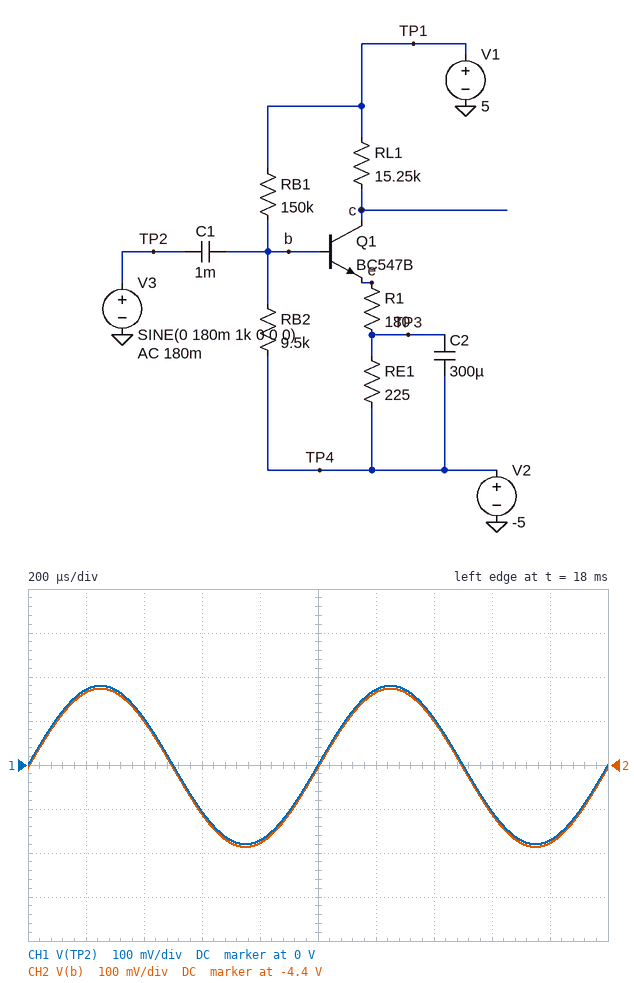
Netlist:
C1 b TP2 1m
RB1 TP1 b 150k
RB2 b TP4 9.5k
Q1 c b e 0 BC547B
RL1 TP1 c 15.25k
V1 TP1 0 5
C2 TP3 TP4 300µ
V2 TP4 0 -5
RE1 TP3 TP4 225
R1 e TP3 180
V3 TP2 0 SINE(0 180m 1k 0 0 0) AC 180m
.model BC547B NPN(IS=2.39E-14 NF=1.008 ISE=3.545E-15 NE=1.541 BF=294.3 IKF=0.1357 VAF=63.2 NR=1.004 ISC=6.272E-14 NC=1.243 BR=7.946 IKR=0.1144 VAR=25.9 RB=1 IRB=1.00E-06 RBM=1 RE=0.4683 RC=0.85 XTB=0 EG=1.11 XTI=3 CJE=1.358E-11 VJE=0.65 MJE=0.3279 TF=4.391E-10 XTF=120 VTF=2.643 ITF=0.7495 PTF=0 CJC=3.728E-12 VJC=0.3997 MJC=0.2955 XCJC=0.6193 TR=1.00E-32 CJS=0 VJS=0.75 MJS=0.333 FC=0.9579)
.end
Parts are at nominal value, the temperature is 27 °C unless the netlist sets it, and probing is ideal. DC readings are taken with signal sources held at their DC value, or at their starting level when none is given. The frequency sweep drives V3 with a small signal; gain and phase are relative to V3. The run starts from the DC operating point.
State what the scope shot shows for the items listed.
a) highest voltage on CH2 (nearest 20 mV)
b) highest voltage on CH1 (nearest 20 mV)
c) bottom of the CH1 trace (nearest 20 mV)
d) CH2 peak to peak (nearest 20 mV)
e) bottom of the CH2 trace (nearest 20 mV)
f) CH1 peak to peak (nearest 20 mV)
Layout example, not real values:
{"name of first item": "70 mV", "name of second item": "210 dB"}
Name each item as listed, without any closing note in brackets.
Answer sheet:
{"highest voltage on CH2": "-4.22 V", "highest voltage on CH1": "180 mV", "bottom of the CH1 trace": "-180 mV", "CH2 peak to peak": "360 mV", "bottom of the CH2 trace": "-4.58 V", "CH1 peak to peak": "360 mV"}
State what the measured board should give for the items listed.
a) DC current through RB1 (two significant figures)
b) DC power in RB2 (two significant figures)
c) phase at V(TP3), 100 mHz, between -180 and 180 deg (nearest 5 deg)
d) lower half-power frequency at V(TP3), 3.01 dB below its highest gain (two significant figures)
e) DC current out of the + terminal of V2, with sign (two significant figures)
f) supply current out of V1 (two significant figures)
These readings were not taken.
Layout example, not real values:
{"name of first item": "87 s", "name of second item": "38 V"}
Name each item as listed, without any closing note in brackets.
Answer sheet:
{"DC current through RB1": "63 µA", "DC power in RB2": "37 µW", "phase at V(TP3), 100 mHz, between -180 and 180 deg": "10 deg", "lower half-power frequency at V(TP3), 3.01 dB below its highest gain": "18 mHz", "DC current out of the + terminal of V2, with sign": "-130 µA", "supply current out of V1": "130 µA"}
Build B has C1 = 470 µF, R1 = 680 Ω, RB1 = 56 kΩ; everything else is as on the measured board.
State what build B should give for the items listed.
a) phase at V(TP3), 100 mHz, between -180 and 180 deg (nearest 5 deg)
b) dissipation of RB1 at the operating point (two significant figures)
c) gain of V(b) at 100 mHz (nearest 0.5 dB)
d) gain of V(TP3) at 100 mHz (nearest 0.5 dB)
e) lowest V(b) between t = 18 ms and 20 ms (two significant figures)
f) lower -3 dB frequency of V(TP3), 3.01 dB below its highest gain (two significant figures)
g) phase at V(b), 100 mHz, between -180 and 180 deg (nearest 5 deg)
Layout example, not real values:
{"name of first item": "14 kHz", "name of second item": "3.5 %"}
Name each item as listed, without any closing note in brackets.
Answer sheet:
{"phase at V(TP3), 100 mHz, between -180 and 180 deg": "70 deg", "dissipation of RB1 at the operating point": "1.4 mW", "gain of V(b) at 100 mHz": "-11.0 dB", "gain of V(TP3) at 100 mHz": "-25.0 dB", "lowest V(b) between t = 18 ms and 20 ms": "-4.0 V", "lower -3 dB frequency of V(TP3), 3.01 dB below its highest gain": "280 mHz", "phase at V(b), 100 mHz, between -180 and 180 deg": "75 deg"}
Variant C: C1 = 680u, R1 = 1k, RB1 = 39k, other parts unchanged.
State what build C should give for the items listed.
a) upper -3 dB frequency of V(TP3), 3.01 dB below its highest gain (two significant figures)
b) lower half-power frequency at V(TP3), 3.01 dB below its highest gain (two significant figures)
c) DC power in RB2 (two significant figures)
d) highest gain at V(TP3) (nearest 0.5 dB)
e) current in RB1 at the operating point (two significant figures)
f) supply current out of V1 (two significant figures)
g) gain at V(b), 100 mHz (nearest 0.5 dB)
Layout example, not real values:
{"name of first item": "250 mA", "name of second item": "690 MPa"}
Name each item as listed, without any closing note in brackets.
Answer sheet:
{"upper -3 dB frequency of V(TP3), 3.01 dB below its highest gain": "3.2 Hz", "lower half-power frequency at V(TP3), 3.01 dB below its highest gain": "180 mHz", "DC power in RB2": "220 µW", "highest gain at V(TP3)": "-16.5 dB", "current in RB1 at the operating point": "220 µA", "supply current out of V1": "820 µA", "gain at V(b), 100 mHz": "-7.0 dB"}
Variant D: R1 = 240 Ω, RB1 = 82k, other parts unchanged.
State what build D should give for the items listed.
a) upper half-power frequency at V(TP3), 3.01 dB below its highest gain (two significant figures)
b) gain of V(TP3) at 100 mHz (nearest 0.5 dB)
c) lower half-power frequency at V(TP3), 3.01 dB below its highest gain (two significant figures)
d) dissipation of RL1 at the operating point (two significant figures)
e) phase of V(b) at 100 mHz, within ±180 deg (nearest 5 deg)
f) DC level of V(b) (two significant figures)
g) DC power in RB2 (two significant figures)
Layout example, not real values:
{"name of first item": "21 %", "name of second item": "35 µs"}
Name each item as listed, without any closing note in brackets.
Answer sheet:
{"upper half-power frequency at V(TP3), 3.01 dB below its highest gain": "4.0 Hz", "gain of V(TP3) at 100 mHz": "-17.5 dB", "lower half-power frequency at V(TP3), 3.01 dB below its highest gain": "190 mHz", "dissipation of RL1 at the operating point": "6.1 mW", "phase of V(b) at 100 mHz, within ±180 deg": "65 deg", "DC level of V(b)": "-4.1 V", "DC power in RB2": "91 µW"}
